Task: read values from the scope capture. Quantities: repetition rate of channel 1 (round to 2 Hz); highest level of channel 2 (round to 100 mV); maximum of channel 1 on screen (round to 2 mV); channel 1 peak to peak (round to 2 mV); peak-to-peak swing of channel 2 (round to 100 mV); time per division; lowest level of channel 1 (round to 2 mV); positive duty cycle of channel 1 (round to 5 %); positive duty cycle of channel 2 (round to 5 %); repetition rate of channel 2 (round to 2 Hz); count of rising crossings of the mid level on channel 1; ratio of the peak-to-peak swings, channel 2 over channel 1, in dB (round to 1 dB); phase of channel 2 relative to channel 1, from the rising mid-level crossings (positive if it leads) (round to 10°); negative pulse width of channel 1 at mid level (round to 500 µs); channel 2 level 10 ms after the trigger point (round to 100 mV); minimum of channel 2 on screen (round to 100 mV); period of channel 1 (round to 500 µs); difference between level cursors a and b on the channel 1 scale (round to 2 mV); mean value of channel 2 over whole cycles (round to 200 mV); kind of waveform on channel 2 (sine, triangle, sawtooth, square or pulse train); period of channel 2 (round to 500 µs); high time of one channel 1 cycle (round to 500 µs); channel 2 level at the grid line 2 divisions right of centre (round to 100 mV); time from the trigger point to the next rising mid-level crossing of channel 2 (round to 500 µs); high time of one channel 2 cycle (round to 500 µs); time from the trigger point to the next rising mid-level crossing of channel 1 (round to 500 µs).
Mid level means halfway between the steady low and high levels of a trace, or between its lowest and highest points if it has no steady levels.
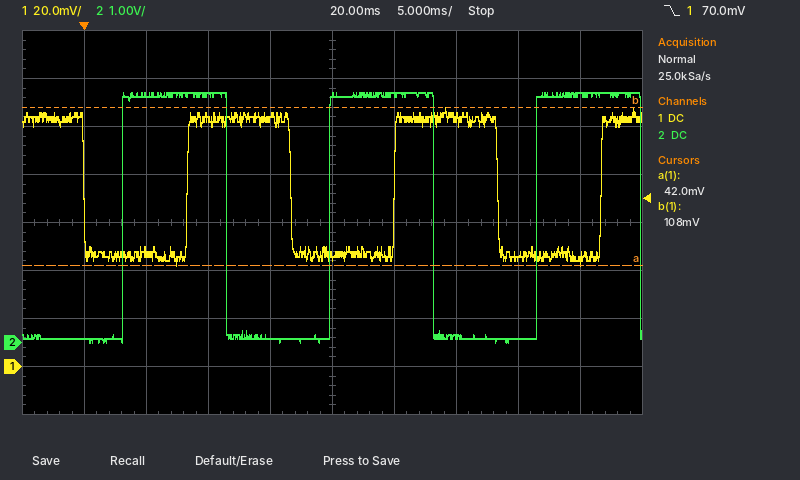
60 Hz
5.2 V
108 mV
66 mV
5.2 V
5 ms
42 mV
50 %
50 %
60 Hz
3
38 dB
+110°
8.5 ms
5.2 V
0.0 V
16.5 ms
66 mV
2.6 V
square
16.5 ms
8.5 ms
100 mV
3.0 ms
8.5 ms
8.5 ms
